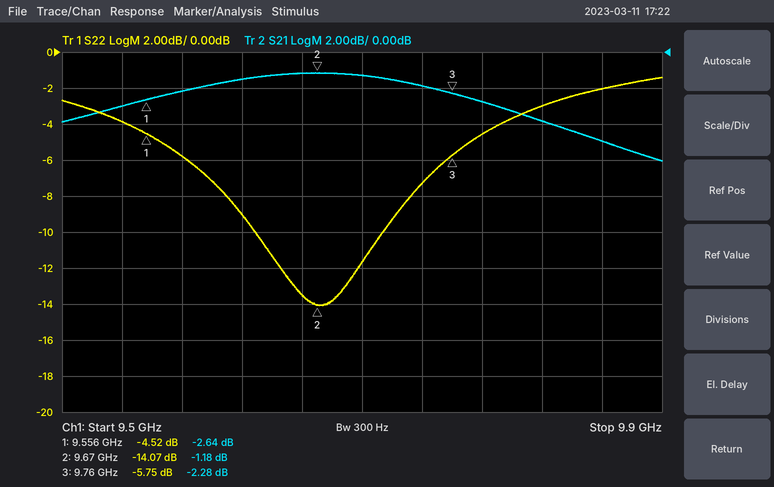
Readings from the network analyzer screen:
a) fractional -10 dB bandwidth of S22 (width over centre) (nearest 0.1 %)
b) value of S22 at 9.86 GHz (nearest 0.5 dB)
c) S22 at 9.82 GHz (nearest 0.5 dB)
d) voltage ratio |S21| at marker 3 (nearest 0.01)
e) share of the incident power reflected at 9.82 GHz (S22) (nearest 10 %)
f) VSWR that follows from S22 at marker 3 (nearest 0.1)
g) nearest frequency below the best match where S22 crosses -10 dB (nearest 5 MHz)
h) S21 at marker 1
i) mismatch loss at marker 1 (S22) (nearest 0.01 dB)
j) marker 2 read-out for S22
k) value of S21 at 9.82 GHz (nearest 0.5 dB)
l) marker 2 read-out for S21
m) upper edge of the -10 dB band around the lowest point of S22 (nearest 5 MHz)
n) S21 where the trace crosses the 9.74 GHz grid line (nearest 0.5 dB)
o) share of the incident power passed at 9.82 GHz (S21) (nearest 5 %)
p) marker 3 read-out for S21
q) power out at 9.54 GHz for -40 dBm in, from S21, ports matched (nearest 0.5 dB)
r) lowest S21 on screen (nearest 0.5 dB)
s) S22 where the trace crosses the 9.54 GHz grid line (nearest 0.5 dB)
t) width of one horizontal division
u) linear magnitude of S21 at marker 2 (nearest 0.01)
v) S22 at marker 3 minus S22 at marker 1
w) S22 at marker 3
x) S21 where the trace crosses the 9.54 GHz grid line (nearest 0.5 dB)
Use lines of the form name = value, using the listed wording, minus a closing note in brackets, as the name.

fractional -10 dB bandwidth of S22 (width over centre) = 0.9 %
value of S22 at 9.86 GHz = -2.0 dB
S22 at 9.82 GHz = -3.0 dB
voltage ratio |S21| at marker 3 = 0.77
share of the incident power reflected at 9.82 GHz (S22) = 50 %
VSWR that follows from S22 at marker 3 = 3.1
nearest frequency below the best match where S22 crosses -10 dB = 9.630 GHz
S21 at marker 1 = -2.64 dB
mismatch loss at marker 1 (S22) = 1.89 dB
marker 2 read-out for S22 = -14.07 dB
value of S21 at 9.82 GHz = -4.0 dB
marker 2 read-out for S21 = -1.18 dB
upper edge of the -10 dB band around the lowest point of S22 = 9.715 GHz
S21 where the trace crosses the 9.74 GHz grid line = -2.0 dB
share of the incident power passed at 9.82 GHz (S21) = 40 %
marker 3 read-out for S21 = -2.28 dB
power out at 9.54 GHz for -40 dBm in, from S21, ports matched = -43.0 dBm
lowest S21 on screen = -6.0 dB
S22 where the trace crosses the 9.54 GHz grid line = -4.0 dB
width of one horizontal division = 40 MHz
linear magnitude of S21 at marker 2 = 0.87
S22 at marker 3 minus S22 at marker 1 = -1.23 dB
S22 at marker 3 = -5.75 dB
S21 where the trace crosses the 9.54 GHz grid line = -3.0 dB
